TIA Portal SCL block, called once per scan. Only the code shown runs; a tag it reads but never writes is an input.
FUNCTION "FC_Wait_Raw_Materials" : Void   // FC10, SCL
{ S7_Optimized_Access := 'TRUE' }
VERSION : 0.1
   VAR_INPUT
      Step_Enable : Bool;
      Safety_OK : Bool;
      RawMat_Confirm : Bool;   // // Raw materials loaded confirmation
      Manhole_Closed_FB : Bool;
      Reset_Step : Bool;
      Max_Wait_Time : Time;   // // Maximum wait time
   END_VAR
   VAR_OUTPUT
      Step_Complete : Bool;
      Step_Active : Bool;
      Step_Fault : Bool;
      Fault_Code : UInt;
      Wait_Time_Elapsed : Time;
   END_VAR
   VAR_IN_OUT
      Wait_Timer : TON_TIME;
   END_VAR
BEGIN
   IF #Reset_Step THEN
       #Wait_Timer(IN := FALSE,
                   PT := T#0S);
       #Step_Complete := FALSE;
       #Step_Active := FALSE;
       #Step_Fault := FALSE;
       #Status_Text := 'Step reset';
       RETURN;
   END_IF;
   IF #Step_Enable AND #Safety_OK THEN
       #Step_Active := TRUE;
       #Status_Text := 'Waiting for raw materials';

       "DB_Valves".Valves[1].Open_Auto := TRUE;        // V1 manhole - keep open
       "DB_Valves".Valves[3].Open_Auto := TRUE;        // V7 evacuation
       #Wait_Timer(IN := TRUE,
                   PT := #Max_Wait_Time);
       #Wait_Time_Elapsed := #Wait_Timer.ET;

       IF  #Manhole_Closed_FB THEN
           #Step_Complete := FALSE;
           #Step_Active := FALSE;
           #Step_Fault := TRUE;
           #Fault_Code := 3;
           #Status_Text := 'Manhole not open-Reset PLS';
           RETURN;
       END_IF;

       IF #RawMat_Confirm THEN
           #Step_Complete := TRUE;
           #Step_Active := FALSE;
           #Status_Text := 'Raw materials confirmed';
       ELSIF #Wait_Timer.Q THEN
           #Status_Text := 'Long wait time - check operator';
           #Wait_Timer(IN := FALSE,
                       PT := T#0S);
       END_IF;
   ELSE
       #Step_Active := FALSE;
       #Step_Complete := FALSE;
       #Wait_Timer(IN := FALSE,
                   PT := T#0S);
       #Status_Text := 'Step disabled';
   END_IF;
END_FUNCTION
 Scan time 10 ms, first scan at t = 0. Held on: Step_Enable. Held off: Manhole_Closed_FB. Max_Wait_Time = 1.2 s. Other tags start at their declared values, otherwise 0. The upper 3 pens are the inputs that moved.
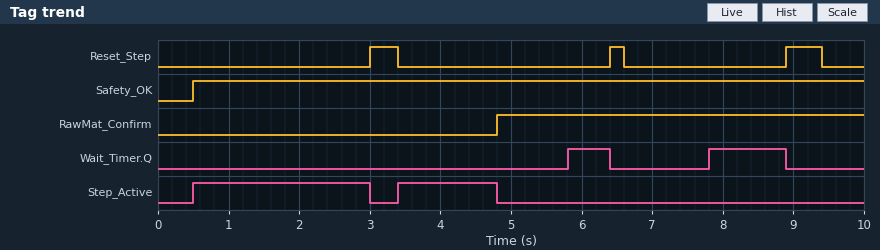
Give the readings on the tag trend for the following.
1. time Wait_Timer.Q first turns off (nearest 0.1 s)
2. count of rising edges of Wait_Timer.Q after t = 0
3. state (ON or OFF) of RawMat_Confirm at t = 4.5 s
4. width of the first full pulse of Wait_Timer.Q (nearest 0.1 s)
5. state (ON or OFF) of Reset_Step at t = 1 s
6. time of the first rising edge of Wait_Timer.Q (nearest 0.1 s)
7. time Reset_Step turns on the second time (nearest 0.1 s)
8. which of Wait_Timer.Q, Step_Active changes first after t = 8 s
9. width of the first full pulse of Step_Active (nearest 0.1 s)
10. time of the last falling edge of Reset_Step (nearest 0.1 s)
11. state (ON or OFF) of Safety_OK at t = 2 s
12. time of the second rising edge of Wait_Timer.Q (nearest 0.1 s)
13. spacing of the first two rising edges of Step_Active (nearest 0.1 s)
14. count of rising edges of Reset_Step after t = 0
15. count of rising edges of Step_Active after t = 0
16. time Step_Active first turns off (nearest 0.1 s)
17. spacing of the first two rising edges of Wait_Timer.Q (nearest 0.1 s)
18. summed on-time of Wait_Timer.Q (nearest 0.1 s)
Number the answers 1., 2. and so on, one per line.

1. 6.4 s
2. 2
3. OFF
4. 0.6 s
5. OFF
6. 5.8 s
7. 6.4 s
8. Wait_Timer.Q
9. 2.5 s
10. 9.4 s
11. ON
12. 7.8 s
13. 2.9 s
14. 3
15. 2
16. 3.0 s
17. 2.0 s
18. 1.7 s
